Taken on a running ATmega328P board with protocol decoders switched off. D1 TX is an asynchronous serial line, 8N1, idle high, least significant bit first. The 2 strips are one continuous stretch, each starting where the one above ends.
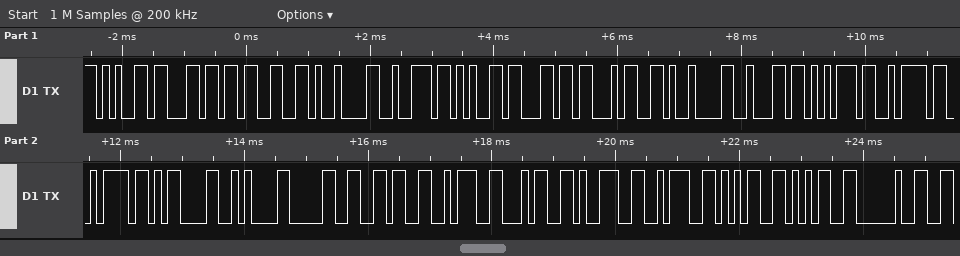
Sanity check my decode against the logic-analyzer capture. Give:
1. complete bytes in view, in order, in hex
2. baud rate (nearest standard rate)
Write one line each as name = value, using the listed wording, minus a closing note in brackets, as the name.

complete bytes in view, in order, in hex = 65 6C 33 09 72 65 6C 34 09 62 75 7A 7A 0D 0A 30 36 3A 34 39 3A 35 35 20
baud rate = 9600 baud
